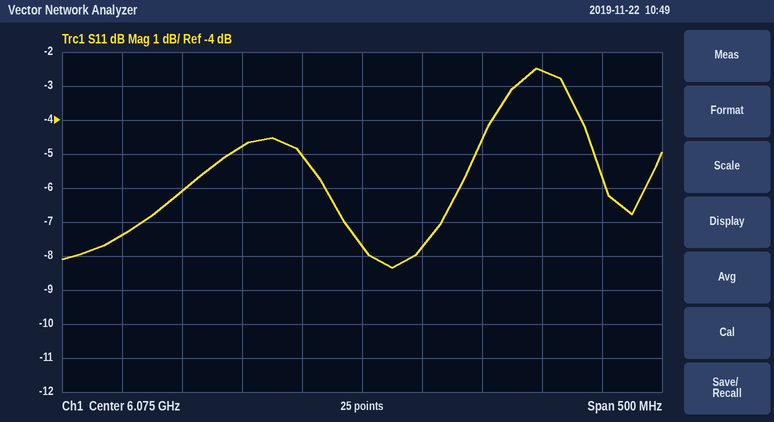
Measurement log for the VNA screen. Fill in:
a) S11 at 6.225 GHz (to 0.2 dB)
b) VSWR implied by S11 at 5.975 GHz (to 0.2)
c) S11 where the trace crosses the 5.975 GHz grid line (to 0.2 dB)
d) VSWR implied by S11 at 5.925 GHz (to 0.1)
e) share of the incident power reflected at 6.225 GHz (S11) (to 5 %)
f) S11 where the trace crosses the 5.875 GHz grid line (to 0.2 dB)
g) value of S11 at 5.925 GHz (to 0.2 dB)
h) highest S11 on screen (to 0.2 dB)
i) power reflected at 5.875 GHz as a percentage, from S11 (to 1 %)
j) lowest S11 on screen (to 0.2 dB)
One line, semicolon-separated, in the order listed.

-2.6 dB; 3.8; -4.8 dB; 3.0; 55 %; -7.4 dB; -6.0 dB; -2.4 dB; 18 %; -8.4 dB
